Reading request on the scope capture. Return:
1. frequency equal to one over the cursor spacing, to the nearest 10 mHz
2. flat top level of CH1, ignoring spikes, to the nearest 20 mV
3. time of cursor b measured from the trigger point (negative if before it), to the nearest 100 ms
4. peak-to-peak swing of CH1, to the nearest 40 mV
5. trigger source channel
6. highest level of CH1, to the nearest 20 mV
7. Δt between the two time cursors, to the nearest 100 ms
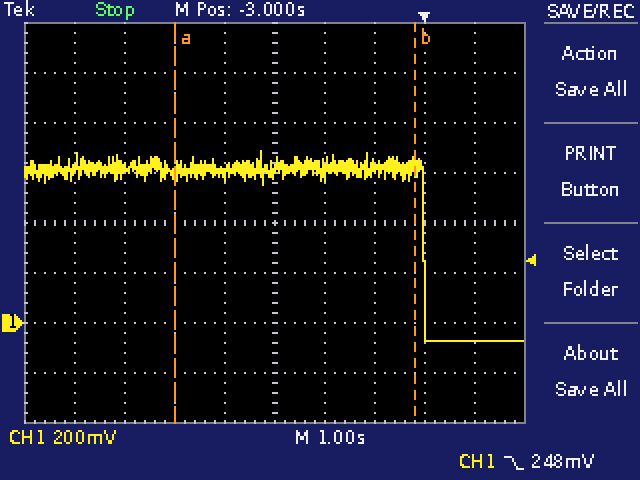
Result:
210 mHz
620 mV
-200 ms
760 mV
CH1
680 mV
4.8 s
